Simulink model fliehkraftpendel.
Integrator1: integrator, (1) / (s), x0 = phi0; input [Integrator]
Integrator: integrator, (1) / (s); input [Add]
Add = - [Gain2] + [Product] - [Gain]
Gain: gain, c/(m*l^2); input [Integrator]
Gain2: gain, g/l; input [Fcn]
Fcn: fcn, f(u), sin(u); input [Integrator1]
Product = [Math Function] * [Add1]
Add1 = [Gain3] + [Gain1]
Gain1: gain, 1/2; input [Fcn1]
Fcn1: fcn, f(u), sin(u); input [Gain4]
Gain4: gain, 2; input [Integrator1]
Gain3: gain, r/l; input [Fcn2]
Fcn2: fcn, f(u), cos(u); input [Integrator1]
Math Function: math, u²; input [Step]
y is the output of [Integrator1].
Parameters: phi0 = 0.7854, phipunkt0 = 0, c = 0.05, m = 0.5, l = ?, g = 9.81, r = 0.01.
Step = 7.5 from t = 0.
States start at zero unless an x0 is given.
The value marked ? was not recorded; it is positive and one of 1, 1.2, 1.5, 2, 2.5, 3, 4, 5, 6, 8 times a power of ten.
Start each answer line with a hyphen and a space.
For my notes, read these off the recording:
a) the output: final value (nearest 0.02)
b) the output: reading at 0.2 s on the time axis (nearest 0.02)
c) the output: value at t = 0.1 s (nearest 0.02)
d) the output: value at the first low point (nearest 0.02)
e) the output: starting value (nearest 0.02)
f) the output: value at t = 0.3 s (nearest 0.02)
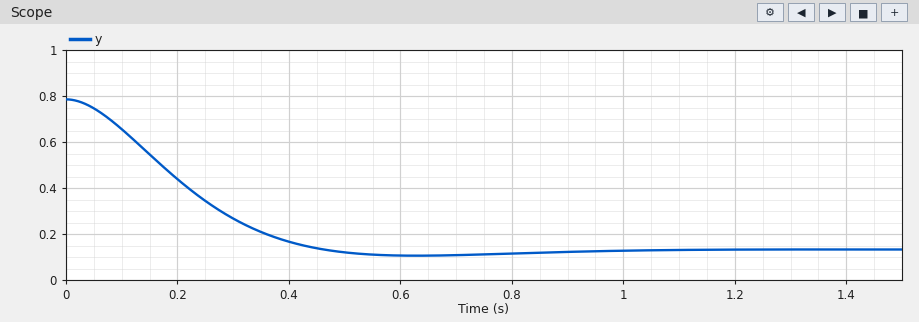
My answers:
- 0.14
- 0.44
- 0.66
- 0.10
- 0.78
- 0.26
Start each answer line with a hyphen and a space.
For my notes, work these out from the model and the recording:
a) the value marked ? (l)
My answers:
- 0.1
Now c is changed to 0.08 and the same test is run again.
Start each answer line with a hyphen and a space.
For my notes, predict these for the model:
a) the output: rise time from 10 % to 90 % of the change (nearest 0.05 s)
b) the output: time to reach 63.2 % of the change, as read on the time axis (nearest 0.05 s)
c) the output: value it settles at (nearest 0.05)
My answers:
- 0.60 s
- 0.30 s
- 0.15
